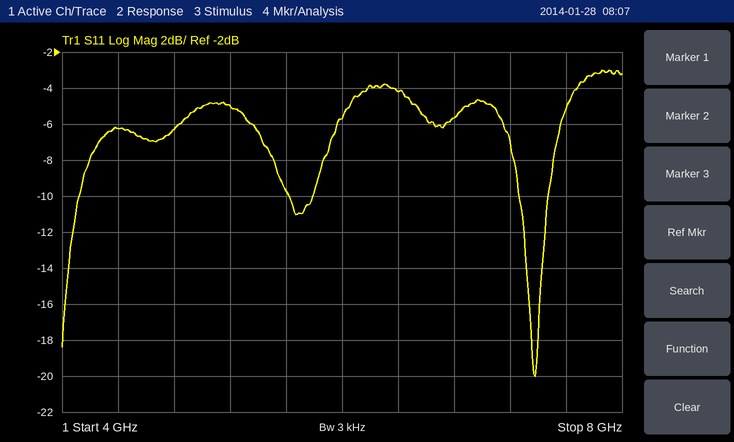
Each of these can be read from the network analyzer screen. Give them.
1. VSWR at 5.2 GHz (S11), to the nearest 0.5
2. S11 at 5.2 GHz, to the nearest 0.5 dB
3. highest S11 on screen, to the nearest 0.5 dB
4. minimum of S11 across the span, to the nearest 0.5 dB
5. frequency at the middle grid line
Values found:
3.5
-5.0 dB
-3.0 dB
-20.0 dB
6 GHz
